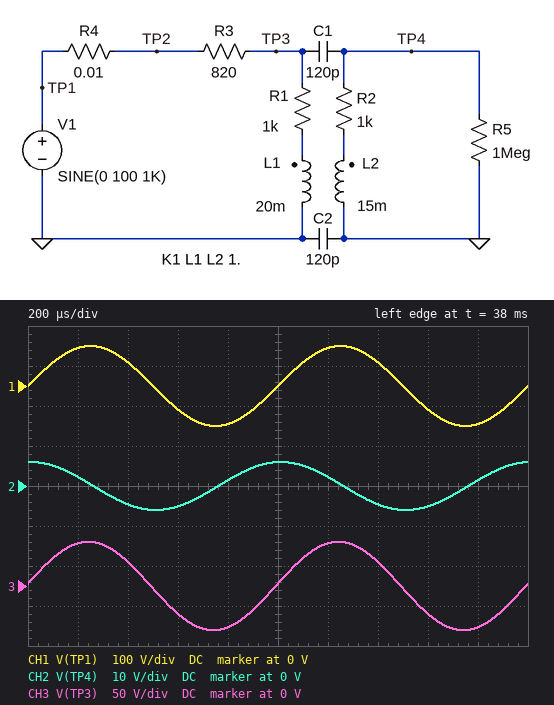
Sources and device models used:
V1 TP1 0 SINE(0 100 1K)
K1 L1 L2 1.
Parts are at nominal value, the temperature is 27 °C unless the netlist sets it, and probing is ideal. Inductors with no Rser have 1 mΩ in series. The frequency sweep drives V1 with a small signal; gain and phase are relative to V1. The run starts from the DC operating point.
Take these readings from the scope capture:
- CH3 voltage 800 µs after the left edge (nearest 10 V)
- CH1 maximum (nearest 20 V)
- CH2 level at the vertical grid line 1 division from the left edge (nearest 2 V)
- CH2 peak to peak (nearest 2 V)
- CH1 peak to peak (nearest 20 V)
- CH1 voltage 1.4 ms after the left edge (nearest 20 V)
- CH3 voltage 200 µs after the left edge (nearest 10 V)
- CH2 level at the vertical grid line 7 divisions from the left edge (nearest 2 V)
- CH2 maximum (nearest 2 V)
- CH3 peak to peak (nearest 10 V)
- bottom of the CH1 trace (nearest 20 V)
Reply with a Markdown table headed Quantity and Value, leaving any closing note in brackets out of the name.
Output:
| Quantity | Value |
|---|---|
| CH3 voltage 800 µs after the left edge | -50 V |
| CH1 maximum | 100 V |
| CH2 level at the vertical grid line 1 division from the left edge | 2 V |
| CH2 peak to peak | 12 V |
| CH1 peak to peak | 200 V |
| CH1 voltage 1.4 ms after the left edge | 60 V |
| CH3 voltage 200 µs after the left edge | 50 V |
| CH2 level at the vertical grid line 7 divisions from the left edge | -4 V |
| CH2 maximum | 6 V |
| CH3 peak to peak | 110 V |
| bottom of the CH1 trace | -100 V |
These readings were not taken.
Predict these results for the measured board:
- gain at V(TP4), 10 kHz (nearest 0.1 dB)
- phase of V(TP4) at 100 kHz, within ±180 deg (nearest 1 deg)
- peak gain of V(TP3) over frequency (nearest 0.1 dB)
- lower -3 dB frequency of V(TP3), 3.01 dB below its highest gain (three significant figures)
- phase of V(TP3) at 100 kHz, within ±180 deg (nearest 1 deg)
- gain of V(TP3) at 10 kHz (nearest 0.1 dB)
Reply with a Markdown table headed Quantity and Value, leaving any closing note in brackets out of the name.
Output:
| Quantity | Value |
|---|---|
| gain at V(TP4), 10 kHz | -6.1 dB |
| phase of V(TP4) at 100 kHz, within ±180 deg | 9 deg |
| peak gain of V(TP3) over frequency | 0 dB |
| lower -3 dB frequency of V(TP3), 3.01 dB below its highest gain | 9.05 kHz |
| phase of V(TP3) at 100 kHz, within ±180 deg | 4 deg |
| gain of V(TP3) at 10 kHz | -2.8 dB |
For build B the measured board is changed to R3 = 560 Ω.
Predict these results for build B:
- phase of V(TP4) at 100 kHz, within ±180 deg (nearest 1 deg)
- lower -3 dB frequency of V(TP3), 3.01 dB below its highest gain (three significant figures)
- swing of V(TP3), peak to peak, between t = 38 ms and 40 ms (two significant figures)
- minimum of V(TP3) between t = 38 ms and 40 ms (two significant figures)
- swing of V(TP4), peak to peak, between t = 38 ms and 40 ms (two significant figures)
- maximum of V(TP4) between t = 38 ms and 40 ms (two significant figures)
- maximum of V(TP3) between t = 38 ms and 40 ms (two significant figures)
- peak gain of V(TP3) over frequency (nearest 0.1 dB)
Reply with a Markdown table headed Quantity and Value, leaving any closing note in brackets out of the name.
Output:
| Quantity | Value |
|---|---|
| phase of V(TP4) at 100 kHz, within ±180 deg | 8 deg |
| lower -3 dB frequency of V(TP3), 3.01 dB below its highest gain | 5.18 kHz |
| swing of V(TP3), peak to peak, between t = 38 ms and 40 ms | 130 V |
| minimum of V(TP3) between t = 38 ms and 40 ms | -64 V |
| swing of V(TP4), peak to peak, between t = 38 ms and 40 ms | 14 V |
| maximum of V(TP4) between t = 38 ms and 40 ms | 7.0 V |
| maximum of V(TP3) between t = 38 ms and 40 ms | 64 V |
| peak gain of V(TP3) over frequency | 0 dB |
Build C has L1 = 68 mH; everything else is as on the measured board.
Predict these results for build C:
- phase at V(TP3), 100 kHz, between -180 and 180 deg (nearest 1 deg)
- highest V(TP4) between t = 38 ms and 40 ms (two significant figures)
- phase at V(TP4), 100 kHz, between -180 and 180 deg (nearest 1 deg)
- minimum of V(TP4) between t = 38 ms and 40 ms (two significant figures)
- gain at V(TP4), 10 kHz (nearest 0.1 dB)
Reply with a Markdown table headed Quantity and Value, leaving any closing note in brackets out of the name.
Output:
| Quantity | Value |
|---|---|
| phase at V(TP3), 100 kHz, between -180 and 180 deg | 1 deg |
| highest V(TP4) between t = 38 ms and 40 ms | 13 V |
| phase at V(TP4), 100 kHz, between -180 and 180 deg | -3 deg |
| minimum of V(TP4) between t = 38 ms and 40 ms | -13 V |
| gain at V(TP4), 10 kHz | 0.5 dB |
